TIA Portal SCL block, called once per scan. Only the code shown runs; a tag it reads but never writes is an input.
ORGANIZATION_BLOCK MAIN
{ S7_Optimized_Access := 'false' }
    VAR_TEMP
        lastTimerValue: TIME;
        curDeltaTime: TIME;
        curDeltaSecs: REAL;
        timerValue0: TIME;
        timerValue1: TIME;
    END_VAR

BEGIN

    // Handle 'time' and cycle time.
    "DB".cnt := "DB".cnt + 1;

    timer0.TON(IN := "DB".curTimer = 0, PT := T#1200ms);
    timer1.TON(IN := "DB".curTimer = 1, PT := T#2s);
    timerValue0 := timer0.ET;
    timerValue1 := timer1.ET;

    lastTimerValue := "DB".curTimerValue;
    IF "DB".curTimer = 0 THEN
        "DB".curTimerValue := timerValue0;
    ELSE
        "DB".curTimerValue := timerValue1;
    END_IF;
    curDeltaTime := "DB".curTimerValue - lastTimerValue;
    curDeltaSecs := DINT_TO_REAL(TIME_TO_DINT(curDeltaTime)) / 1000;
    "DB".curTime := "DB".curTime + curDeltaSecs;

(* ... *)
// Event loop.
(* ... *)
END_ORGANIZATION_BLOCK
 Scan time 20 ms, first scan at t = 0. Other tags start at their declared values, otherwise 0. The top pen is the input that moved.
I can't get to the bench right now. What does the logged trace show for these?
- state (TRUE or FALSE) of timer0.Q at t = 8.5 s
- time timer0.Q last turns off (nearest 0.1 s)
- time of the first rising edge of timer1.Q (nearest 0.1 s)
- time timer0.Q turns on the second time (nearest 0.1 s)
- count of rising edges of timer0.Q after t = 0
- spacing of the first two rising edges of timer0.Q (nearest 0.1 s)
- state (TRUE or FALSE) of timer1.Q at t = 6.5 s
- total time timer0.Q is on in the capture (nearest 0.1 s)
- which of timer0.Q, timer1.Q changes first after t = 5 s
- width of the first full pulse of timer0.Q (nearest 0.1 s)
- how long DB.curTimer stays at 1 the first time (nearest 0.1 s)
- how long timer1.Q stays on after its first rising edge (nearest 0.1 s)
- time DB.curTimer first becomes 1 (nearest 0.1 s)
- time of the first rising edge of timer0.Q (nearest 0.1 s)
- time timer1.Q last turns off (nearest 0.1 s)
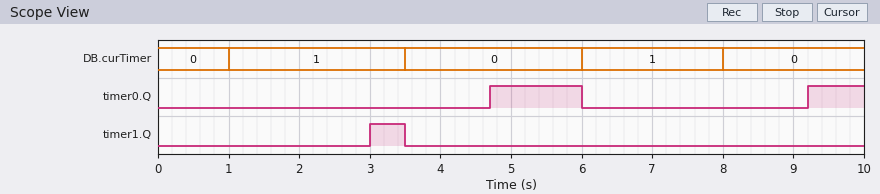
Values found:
FALSE
6.0 s
3.0 s
9.2 s
2
4.5 s
FALSE
2.1 s
timer0.Q
1.3 s
2.5 s
0.5 s
1.0 s
4.7 s
3.5 s
